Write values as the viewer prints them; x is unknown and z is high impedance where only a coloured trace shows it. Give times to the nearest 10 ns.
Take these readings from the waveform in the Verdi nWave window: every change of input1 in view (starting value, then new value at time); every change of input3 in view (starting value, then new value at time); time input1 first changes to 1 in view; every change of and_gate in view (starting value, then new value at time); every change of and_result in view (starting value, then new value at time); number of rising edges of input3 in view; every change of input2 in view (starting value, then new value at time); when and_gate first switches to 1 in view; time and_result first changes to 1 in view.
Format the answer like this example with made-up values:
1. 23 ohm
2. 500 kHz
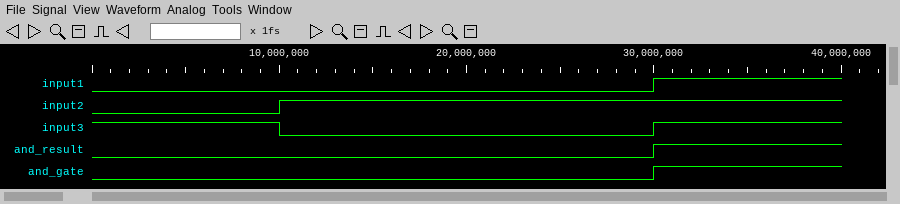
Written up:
1. 0, 1 at 30 ns
2. 1, 0 at 10 ns, 1 at 30 ns
3. 30 ns
4. 0, 1 at 30 ns
5. 0, 1 at 30 ns
6. 1
7. 0, 1 at 10 ns
8. 30 ns
9. 30 ns
